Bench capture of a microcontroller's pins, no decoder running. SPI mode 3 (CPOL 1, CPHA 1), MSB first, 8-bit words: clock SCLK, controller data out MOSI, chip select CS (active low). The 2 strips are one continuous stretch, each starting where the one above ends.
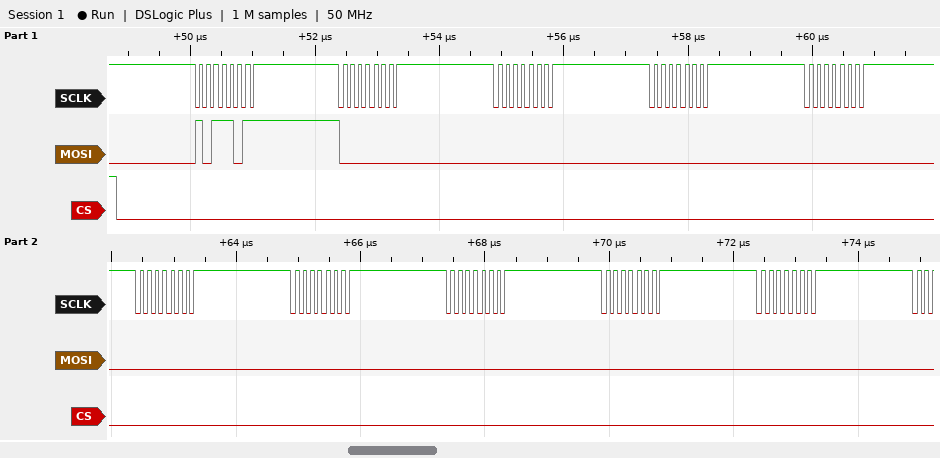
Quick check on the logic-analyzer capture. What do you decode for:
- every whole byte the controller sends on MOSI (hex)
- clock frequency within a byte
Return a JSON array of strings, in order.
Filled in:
["0xBB 0x00 0x00 0x00 0x00 0x00 0x00 0x00 0x00 0x00", "8 MHz"]
